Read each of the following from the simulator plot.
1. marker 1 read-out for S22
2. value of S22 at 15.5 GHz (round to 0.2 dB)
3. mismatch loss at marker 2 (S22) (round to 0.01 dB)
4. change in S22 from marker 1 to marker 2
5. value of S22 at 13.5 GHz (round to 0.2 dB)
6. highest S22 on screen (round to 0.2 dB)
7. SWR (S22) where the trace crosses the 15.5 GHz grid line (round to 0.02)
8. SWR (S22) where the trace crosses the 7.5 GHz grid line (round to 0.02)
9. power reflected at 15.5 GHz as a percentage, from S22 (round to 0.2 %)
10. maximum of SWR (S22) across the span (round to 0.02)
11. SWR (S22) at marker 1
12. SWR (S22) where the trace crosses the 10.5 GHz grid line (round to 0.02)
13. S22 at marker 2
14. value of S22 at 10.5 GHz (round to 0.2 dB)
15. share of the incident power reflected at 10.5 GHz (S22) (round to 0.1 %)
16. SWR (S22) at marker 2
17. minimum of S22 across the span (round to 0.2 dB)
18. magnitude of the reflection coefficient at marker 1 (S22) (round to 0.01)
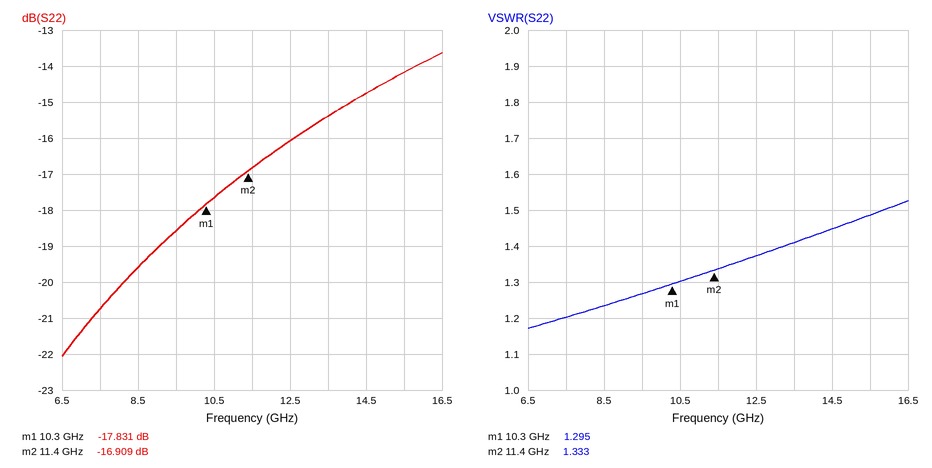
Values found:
-17.831 dB
-14.2 dB
0.09 dB
0.922 dB
-15.4 dB
-13.6 dB
1.48
1.20
3.8 %
1.52
1.295
1.30
-16.909 dB
-17.6 dB
1.7 %
1.333
-22.0 dB
0.13
